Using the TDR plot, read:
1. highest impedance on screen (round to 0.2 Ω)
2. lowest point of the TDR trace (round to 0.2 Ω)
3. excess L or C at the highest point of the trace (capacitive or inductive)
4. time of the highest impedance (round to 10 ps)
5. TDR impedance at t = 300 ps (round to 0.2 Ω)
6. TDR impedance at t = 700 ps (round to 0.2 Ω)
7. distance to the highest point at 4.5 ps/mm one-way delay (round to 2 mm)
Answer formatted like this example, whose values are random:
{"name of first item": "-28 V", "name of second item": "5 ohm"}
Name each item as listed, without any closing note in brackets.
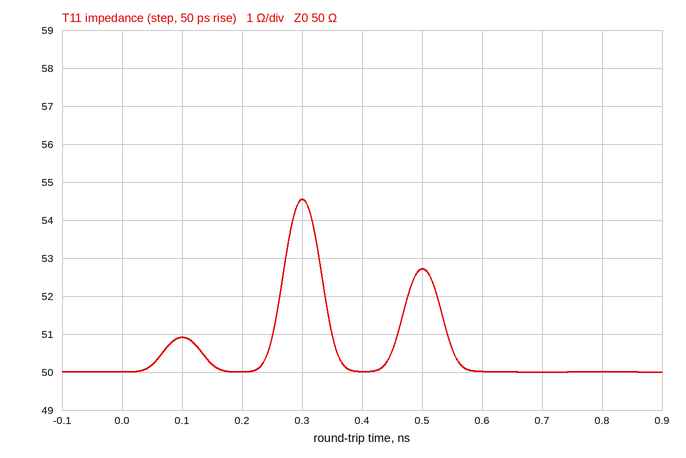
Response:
{"highest impedance on screen": "54.6 Ω", "lowest point of the TDR trace": "50.0 Ω", "excess L or C at the highest point of the trace": "inductive", "time of the highest impedance": "300 ps", "TDR impedance at t = 300 ps": "54.6 Ω", "TDR impedance at t = 700 ps": "50.0 Ω", "distance to the highest point at 4.5 ps/mm one-way delay": "34 mm"}
